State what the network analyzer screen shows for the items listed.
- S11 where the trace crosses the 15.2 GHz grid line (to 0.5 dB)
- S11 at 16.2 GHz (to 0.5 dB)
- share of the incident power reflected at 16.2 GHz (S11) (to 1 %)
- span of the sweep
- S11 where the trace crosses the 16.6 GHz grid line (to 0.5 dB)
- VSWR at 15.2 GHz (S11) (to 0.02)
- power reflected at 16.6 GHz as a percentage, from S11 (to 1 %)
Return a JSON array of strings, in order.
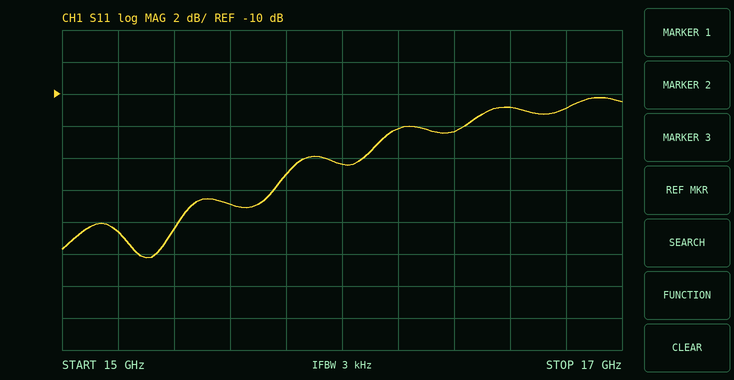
["-18.5 dB", "-12.0 dB", "6 %", "2 GHz", "-11.0 dB", "1.26", "8 %"]
